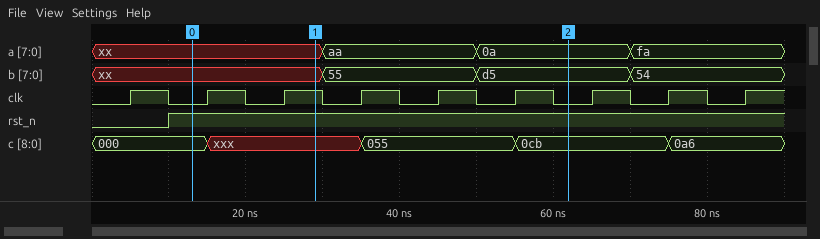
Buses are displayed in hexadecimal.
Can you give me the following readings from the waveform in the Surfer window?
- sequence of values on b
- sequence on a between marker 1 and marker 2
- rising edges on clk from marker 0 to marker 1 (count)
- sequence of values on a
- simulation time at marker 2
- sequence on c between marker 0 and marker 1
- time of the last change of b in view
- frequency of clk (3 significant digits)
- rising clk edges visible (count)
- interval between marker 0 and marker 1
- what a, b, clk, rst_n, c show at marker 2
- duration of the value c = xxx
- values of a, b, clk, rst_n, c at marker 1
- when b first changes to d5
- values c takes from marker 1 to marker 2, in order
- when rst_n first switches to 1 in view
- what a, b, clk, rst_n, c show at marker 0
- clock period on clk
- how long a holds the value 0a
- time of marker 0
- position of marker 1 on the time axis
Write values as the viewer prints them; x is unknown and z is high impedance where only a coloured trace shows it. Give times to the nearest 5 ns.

xx, 55, d5, 54
xx, aa, 0a
2
xx, aa, 0a, fa
60 ns
000, xxx
70 ns
100 MHz
9
15 ns
a=0a, b=d5, clk=0, rst_n=1, c=0cb
20 ns
a=xx, b=xx, clk=1, rst_n=1, c=xxx
50 ns
xxx, 055, 0cb
10 ns
a=xx, b=xx, clk=0, rst_n=1, c=000
10 ns
20 ns
15 ns
30 ns
